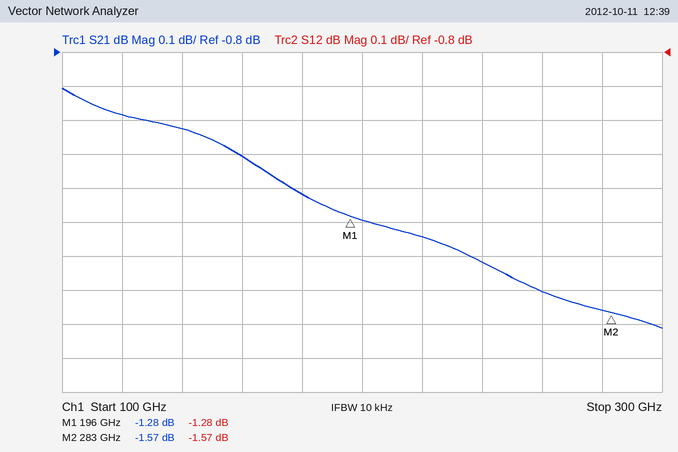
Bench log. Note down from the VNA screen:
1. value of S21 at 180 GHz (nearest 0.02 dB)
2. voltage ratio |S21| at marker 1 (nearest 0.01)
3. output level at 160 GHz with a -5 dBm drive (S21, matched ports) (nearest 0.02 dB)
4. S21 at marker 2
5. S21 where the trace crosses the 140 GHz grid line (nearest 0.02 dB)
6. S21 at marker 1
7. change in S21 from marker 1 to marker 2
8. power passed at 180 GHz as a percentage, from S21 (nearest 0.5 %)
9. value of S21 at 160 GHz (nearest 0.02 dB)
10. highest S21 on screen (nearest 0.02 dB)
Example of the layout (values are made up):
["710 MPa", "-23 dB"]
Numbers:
["-1.22 dB", "0.86", "-6.10 dBm", "-1.57 dB", "-1.02 dB", "-1.28 dB", "-0.29 dB", "75.5 %", "-1.10 dB", "-0.90 dB"]
